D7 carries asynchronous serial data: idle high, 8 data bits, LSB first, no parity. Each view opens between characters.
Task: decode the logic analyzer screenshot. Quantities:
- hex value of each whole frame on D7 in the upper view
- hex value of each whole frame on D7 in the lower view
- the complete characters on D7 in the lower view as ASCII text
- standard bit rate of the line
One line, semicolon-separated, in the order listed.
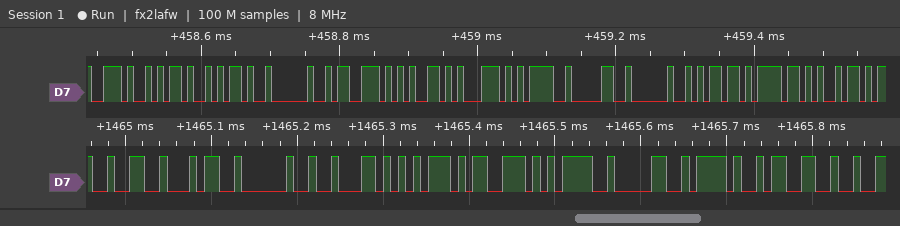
2E, 2D, 2D, 20, 73, 65, 71, 3D, 30, 20, 6D, 6F, 69; 32, 34, 20, 62, 75, 73, 3D, 30, 2F, 33; "24 bus=0/3"; 115200 baud
